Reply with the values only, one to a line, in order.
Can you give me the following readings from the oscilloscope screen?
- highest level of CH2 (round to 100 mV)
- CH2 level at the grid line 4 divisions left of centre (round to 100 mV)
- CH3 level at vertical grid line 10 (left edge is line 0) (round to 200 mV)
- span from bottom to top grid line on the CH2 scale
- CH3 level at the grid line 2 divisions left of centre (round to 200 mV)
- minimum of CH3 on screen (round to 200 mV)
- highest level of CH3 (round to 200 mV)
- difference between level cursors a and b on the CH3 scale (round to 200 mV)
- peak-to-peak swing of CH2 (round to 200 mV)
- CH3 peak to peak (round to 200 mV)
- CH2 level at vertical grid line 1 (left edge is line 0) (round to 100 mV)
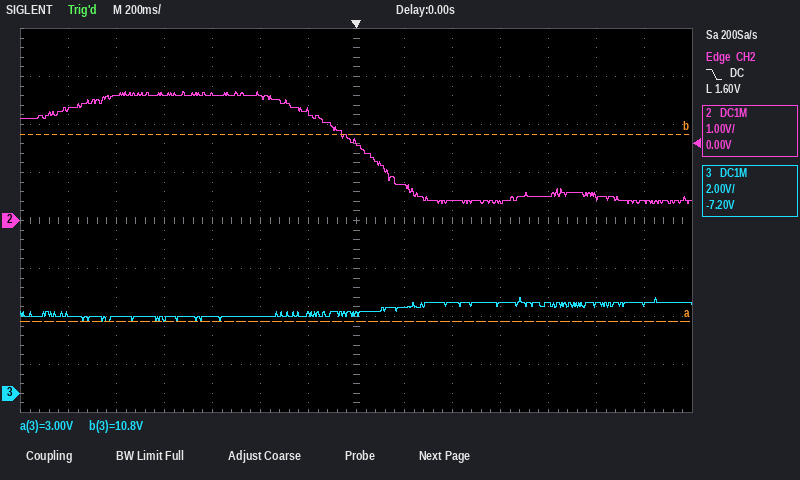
2.7 V
2.6 V
3.8 V
8 V
3.2 V
3.0 V
4.0 V
7.8 V
2.4 V
1.0 V
2.3 V
